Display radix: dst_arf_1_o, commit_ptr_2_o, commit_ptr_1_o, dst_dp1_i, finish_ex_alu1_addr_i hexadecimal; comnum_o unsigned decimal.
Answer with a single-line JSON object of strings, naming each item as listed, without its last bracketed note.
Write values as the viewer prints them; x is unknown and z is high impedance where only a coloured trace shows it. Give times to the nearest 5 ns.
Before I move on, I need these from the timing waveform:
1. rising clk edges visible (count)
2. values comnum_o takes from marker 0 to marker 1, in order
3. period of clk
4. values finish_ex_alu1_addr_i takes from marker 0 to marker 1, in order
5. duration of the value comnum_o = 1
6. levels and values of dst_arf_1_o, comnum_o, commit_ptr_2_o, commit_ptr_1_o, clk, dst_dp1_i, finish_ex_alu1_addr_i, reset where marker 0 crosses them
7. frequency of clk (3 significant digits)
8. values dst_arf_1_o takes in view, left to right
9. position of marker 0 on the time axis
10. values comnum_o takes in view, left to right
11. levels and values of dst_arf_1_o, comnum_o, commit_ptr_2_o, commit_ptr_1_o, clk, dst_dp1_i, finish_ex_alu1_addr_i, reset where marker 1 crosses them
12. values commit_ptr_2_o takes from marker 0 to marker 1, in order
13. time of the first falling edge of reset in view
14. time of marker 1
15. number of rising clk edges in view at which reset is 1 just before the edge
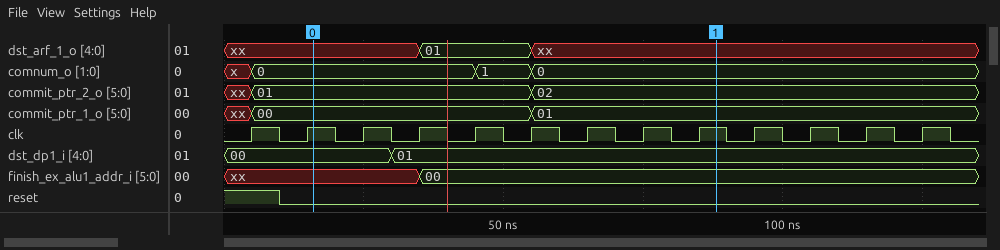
{"rising clk edges visible": "13", "values comnum_o takes from marker 0 to marker 1, in order": "0, 1, 0", "period of clk": "10 ns", "values finish_ex_alu1_addr_i takes from marker 0 to marker 1, in order": "xx, 00", "duration of the value comnum_o = 1": "10 ns", "levels and values of dst_arf_1_o, comnum_o, commit_ptr_2_o, commit_ptr_1_o, clk, dst_dp1_i, finish_ex_alu1_addr_i, reset where marker 0 crosses them": "dst_arf_1_o=xx, comnum_o=0, commit_ptr_2_o=01, commit_ptr_1_o=00, clk=1, dst_dp1_i=00, finish_ex_alu1_addr_i=xx, reset=0", "frequency of clk": "100 MHz", "values dst_arf_1_o takes in view, left to right": "xx, 01, xx", "position of marker 0 on the time axis": "15 ns", "values comnum_o takes in view, left to right": "x, 0, 1, 0", "levels and values of dst_arf_1_o, comnum_o, commit_ptr_2_o, commit_ptr_1_o, clk, dst_dp1_i, finish_ex_alu1_addr_i, reset where marker 1 crosses them": "dst_arf_1_o=xx, comnum_o=0, commit_ptr_2_o=02, commit_ptr_1_o=01, clk=1, dst_dp1_i=01, finish_ex_alu1_addr_i=00, reset=0", "values commit_ptr_2_o takes from marker 0 to marker 1, in order": "01, 02", "time of the first falling edge of reset in view": "10 ns", "time of marker 1": "90 ns", "number of rising clk edges in view at which reset is 1 just before the edge": "1"}
